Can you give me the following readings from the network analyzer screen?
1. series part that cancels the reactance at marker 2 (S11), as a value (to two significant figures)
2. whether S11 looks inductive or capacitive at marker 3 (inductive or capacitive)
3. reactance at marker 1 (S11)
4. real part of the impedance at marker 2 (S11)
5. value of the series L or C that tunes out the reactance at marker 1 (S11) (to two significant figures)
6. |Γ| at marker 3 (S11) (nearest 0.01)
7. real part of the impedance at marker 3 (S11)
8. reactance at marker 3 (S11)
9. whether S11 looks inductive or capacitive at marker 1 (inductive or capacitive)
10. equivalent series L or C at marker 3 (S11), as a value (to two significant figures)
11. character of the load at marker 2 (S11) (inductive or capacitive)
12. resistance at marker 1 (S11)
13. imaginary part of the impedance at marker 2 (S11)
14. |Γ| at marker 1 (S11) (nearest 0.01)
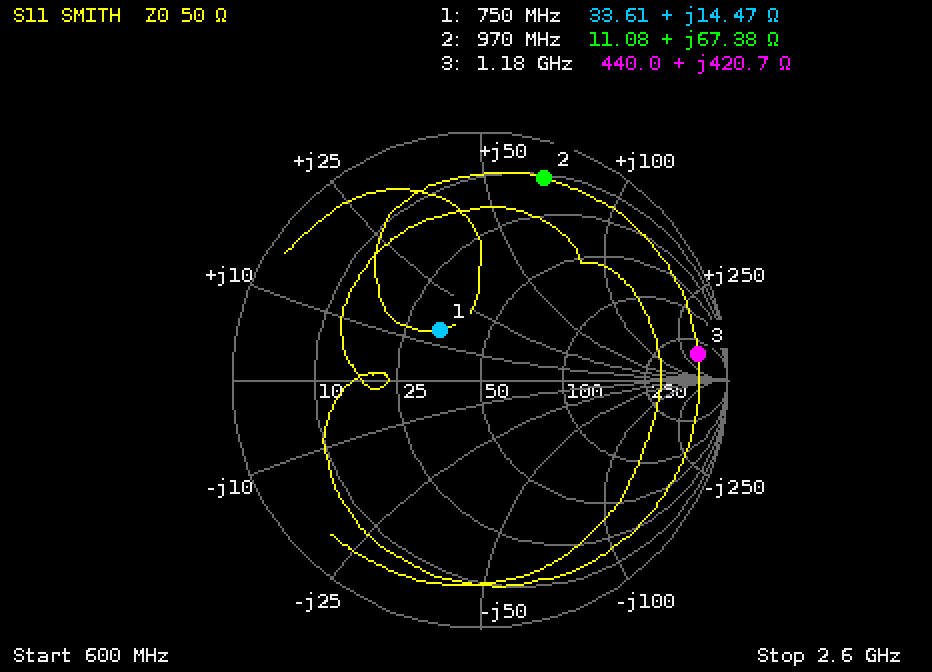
2.4 pF
inductive
+14.47 Ω
11.08 Ω
15 pF
0.89
440.0 Ω
+420.7 Ω
inductive
57 nH
inductive
33.61 Ω
+67.38 Ω
0.26
